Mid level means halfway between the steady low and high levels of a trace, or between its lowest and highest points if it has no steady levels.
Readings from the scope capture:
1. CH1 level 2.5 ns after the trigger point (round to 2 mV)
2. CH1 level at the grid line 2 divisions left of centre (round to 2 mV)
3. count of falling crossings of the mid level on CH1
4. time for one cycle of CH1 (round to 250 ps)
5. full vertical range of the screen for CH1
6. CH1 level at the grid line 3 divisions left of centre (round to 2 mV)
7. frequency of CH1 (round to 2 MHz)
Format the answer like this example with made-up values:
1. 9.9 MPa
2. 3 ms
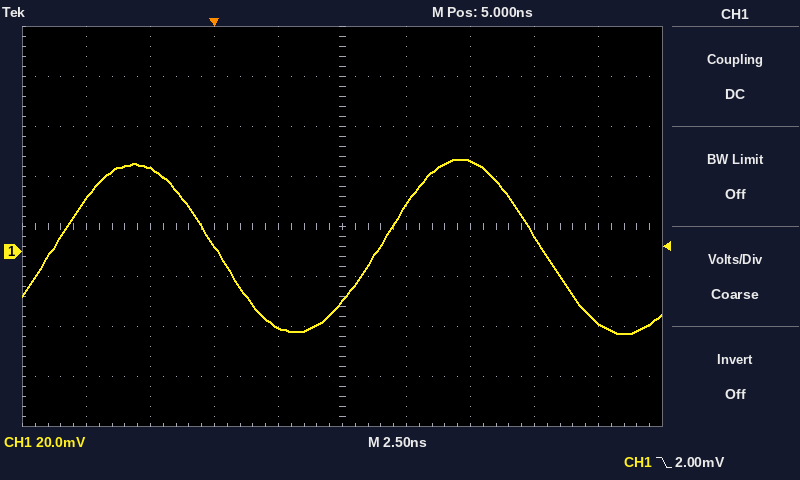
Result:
1. -30 mV
2. 2 mV
3. 2
4. 12.75 ns
5. 160 mV
6. 34 mV
7. 78 MHz
